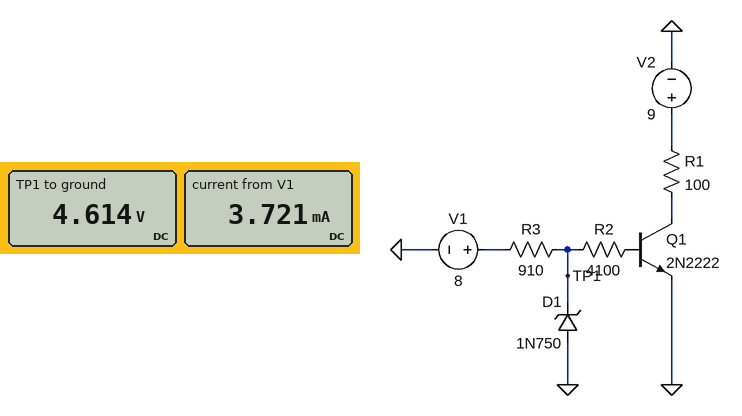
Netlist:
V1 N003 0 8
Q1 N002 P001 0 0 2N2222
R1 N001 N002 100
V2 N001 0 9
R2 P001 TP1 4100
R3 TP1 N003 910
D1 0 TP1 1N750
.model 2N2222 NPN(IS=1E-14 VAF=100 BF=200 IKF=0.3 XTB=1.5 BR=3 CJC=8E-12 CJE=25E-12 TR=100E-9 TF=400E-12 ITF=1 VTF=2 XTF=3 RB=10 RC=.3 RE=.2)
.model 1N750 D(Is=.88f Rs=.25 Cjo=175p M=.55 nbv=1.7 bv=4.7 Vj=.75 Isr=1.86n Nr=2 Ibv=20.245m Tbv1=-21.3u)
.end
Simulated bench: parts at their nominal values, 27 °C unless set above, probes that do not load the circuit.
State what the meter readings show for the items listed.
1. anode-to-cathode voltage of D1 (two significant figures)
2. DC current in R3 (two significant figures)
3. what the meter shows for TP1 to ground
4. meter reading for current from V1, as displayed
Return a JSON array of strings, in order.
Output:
["-4.6 V", "3.7 mA", "4.614 V", "3.721 mA"]
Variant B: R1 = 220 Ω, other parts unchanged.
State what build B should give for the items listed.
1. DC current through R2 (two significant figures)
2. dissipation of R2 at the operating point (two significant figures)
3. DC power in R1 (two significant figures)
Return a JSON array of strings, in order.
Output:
["940 µA", "3.6 mW", "360 mW"]
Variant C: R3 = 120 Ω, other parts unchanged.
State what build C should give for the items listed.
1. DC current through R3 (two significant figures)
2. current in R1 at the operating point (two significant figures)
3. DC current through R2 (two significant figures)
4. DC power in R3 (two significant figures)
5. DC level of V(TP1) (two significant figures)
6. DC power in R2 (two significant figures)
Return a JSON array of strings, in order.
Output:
["27 mA", "88 mA", "950 µA", "90 mW", "4.7 V", "3.7 mW"]
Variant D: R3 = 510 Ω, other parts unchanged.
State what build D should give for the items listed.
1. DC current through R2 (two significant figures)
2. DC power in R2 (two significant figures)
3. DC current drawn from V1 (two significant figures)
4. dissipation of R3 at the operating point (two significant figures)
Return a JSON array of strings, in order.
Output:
["940 µA", "3.6 mW", "6.6 mA", "22 mW"]
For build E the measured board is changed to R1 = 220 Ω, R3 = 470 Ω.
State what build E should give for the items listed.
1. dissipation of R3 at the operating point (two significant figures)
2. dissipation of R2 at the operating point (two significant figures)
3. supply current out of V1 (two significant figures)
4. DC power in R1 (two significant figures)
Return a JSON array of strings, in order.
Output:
["24 mW", "3.7 mW", "7.1 mA", "360 mW"]
